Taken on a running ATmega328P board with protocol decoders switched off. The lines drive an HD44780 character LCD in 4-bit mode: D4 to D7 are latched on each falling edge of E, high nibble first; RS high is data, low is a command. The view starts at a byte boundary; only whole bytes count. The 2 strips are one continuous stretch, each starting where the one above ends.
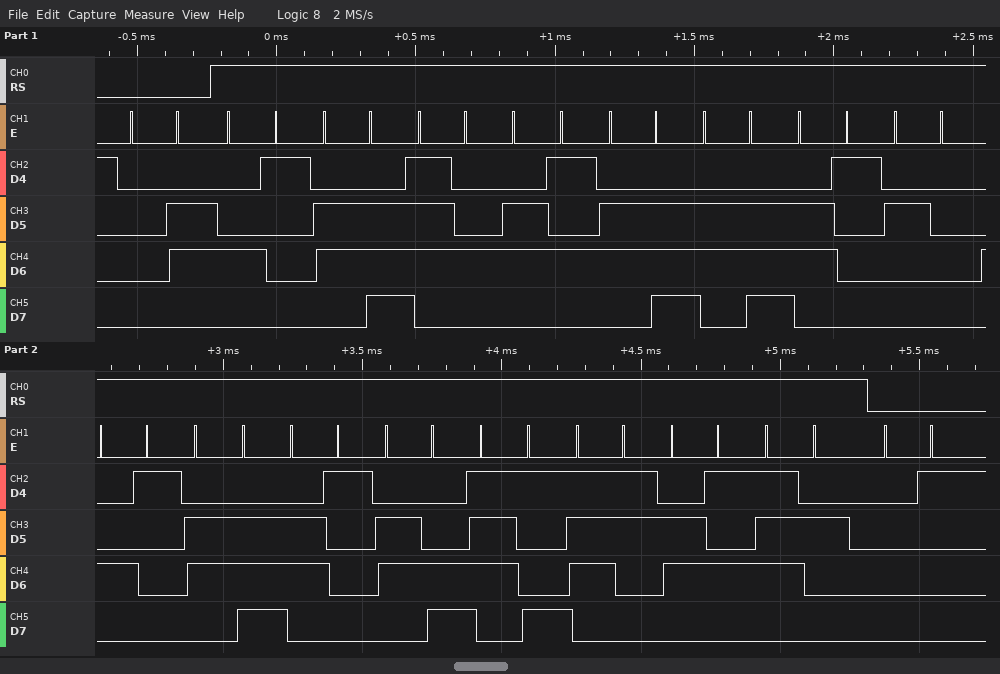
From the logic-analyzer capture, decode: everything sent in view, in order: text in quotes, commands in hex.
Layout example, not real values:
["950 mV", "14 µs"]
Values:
["0x06 \"Antenna Analyser\" 0x01"]
